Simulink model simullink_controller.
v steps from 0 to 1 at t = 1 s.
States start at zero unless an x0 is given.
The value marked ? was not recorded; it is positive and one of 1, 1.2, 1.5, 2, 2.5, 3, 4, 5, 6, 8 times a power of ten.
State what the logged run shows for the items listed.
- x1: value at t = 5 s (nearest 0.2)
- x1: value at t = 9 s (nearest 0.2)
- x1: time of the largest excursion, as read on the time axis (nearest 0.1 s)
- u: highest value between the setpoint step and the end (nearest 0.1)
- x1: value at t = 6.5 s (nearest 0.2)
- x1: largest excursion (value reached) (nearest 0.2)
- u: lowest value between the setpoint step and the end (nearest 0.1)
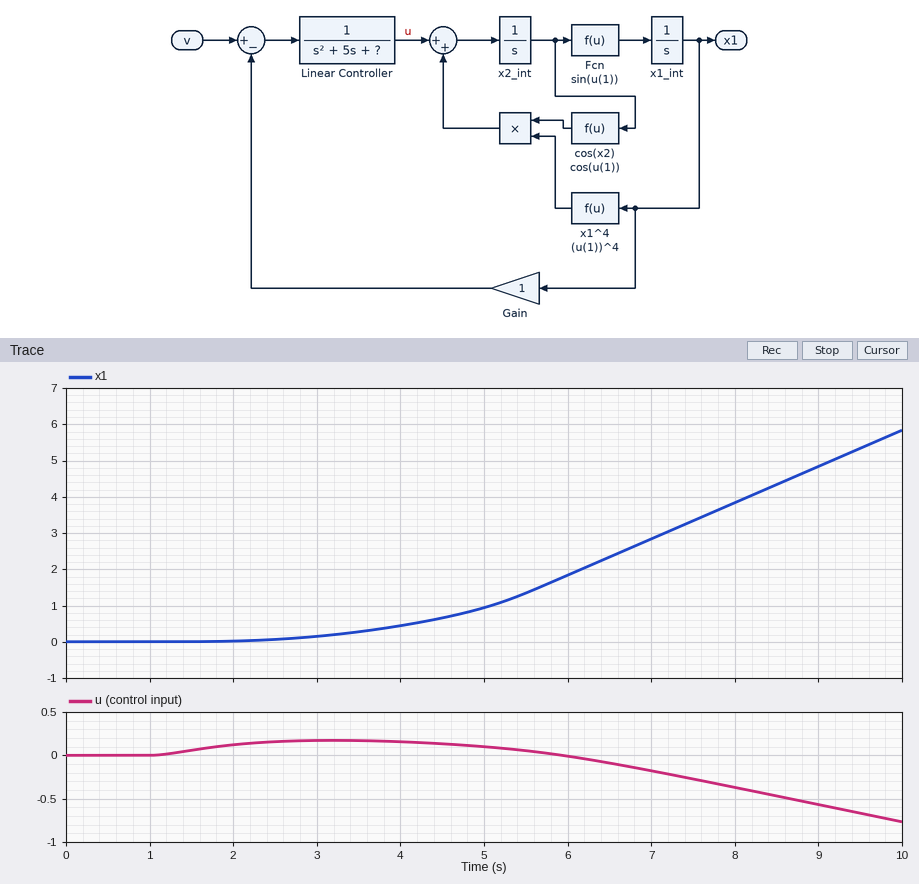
1.0
4.8
10.0 s
0.2
2.4
5.8
-0.8
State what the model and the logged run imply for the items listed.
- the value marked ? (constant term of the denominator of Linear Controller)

5
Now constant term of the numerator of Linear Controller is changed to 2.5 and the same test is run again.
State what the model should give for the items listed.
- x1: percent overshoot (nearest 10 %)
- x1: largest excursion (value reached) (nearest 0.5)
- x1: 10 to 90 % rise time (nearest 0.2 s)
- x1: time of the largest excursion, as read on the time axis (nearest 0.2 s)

110 %
7.0
3.0 s
10.0 s
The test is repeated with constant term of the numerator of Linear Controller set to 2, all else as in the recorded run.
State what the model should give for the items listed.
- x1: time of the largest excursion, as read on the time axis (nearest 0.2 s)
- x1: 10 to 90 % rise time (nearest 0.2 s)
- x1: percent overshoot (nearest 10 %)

10.0 s
3.2 s
100 %
